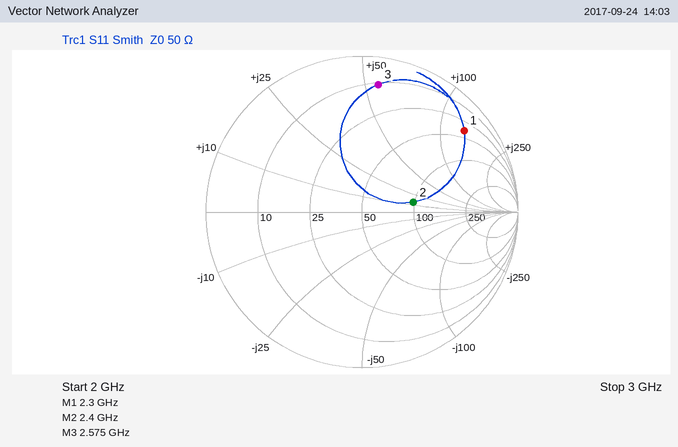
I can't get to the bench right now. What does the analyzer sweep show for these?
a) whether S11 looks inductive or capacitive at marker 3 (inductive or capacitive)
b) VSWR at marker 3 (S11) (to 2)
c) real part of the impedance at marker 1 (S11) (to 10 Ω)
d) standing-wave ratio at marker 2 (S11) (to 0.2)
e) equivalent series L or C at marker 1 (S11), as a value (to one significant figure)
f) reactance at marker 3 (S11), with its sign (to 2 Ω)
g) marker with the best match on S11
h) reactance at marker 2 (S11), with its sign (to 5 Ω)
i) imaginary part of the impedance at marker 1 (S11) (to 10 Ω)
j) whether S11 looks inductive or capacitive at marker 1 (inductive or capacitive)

inductive
10
40 Ω
2.0
9 nH
+56 Ω
marker 2
+15 Ω
+130 Ω
inductive
